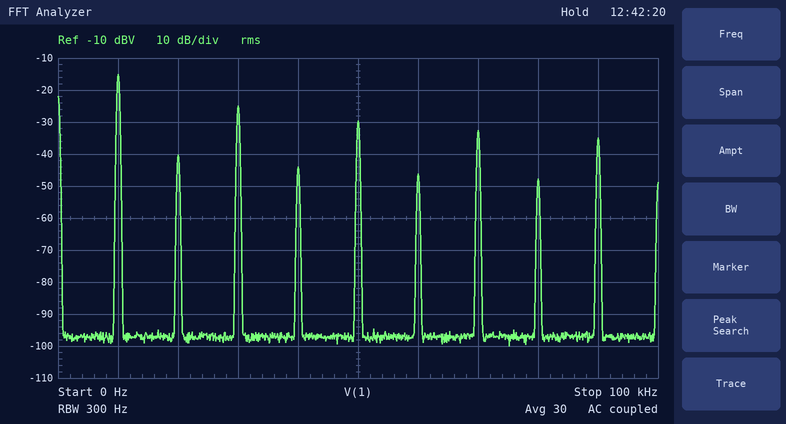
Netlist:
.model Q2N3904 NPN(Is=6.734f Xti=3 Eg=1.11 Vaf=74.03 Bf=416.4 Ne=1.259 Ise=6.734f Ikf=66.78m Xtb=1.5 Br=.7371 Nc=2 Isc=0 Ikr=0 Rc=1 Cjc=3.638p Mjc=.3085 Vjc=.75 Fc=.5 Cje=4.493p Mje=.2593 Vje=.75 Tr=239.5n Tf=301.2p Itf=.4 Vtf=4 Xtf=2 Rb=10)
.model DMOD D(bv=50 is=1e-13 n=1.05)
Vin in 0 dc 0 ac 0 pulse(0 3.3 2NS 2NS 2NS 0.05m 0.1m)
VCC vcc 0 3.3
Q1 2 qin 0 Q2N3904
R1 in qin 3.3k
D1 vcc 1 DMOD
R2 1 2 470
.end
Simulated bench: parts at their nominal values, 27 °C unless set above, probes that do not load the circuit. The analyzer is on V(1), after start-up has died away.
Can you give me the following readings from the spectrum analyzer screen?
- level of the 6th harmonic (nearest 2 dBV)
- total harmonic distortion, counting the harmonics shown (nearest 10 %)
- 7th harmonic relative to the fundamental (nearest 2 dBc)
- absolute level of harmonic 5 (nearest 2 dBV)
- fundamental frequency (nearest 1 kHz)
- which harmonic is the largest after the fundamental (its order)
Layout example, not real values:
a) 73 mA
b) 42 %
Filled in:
a) -46 dBV
b) 40 %
c) -18 dBc
d) -30 dBV
e) 10 kHz
f) 3
